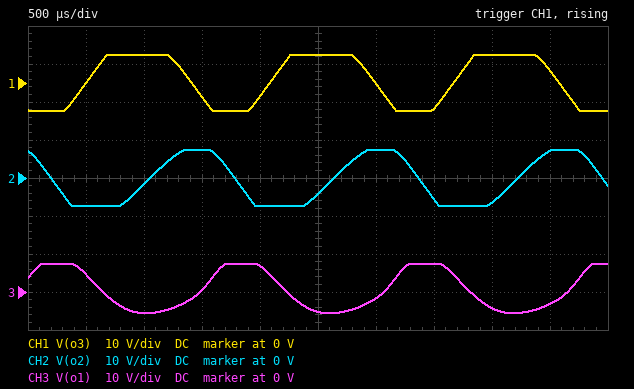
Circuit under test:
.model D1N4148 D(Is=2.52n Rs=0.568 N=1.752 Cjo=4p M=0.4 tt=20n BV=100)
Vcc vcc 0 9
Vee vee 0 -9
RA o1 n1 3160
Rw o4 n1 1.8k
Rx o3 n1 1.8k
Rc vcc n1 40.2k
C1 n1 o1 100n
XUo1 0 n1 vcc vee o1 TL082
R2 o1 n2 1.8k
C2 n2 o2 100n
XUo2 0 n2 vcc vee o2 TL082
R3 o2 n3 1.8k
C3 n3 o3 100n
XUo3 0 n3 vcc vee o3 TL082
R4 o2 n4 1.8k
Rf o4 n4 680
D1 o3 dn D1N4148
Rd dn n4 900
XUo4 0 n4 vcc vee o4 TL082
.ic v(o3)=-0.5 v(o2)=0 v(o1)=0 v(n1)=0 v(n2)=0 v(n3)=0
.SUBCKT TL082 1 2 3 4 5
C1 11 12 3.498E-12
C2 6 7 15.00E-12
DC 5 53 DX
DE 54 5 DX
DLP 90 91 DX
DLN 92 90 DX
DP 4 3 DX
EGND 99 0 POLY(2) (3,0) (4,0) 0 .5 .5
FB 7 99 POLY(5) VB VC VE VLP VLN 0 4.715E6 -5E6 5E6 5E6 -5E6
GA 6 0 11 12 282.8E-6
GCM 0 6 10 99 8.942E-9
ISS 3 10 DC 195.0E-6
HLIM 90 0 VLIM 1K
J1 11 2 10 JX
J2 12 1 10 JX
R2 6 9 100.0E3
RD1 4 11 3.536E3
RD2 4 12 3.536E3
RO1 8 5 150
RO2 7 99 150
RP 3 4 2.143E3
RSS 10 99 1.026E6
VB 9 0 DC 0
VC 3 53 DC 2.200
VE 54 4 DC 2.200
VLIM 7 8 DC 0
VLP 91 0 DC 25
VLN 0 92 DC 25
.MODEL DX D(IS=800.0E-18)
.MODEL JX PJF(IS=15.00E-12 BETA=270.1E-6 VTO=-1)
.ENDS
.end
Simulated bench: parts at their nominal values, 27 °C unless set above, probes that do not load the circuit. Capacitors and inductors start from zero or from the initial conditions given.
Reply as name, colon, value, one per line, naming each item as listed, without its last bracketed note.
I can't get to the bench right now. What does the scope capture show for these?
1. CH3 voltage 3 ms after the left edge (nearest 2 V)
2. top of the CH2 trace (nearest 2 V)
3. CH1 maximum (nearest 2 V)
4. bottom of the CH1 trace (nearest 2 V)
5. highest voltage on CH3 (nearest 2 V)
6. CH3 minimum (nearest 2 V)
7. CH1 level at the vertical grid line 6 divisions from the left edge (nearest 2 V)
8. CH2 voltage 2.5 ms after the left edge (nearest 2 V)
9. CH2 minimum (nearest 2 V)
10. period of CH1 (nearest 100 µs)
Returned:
CH3 voltage 3 ms after the left edge: -2 V
top of the CH2 trace: 8 V
CH1 maximum: 8 V
bottom of the CH1 trace: -8 V
highest voltage on CH3: 8 V
CH3 minimum: -6 V
CH1 level at the vertical grid line 6 divisions from the left edge: 0 V
CH2 voltage 2.5 ms after the left edge: -4 V
CH2 minimum: -8 V
period of CH1: 1.6 ms
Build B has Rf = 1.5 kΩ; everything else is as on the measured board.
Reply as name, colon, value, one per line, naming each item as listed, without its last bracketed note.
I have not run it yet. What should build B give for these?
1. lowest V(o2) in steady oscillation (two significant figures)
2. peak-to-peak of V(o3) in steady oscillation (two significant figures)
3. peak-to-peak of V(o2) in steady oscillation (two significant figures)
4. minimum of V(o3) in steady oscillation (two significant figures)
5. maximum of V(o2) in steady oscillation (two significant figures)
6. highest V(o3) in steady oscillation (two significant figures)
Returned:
lowest V(o2) in steady oscillation: -2.2 V
peak-to-peak of V(o3) in steady oscillation: 4.7 V
peak-to-peak of V(o2) in steady oscillation: 3.7 V
minimum of V(o3) in steady oscillation: -2.0 V
maximum of V(o2) in steady oscillation: 1.5 V
highest V(o3) in steady oscillation: 2.7 V
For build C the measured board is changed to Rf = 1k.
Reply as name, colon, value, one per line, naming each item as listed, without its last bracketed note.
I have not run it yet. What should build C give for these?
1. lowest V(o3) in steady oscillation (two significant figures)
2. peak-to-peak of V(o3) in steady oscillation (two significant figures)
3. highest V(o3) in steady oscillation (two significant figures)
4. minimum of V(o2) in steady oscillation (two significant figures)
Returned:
lowest V(o3) in steady oscillation: -3.1 V
peak-to-peak of V(o3) in steady oscillation: 10 V
highest V(o3) in steady oscillation: 7.3 V
minimum of V(o2) in steady oscillation: -4.2 V
